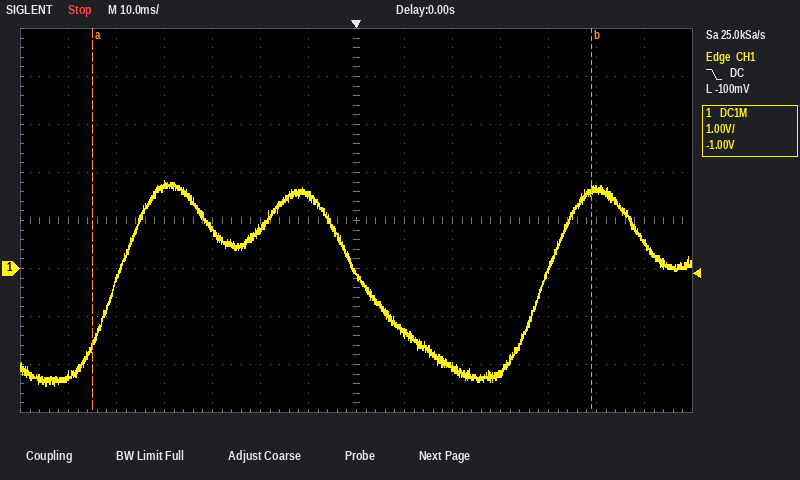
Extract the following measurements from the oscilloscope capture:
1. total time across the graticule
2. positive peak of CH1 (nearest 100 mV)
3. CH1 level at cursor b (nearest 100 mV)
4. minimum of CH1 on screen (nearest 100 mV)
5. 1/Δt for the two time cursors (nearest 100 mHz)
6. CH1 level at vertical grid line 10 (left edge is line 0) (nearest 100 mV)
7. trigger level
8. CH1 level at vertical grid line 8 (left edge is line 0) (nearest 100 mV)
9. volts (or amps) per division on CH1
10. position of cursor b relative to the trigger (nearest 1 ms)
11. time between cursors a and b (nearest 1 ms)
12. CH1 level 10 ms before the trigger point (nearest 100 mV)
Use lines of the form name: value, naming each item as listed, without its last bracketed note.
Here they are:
total time across the graticule: 140 ms
positive peak of CH1: 1.8 V
CH1 level at cursor b: 1.6 V
minimum of CH1 on screen: -2.4 V
1/Δt for the two time cursors: 9.6 Hz
CH1 level at vertical grid line 10 (left edge is line 0): -2.2 V
trigger level: -100 mV
CH1 level at vertical grid line 8 (left edge is line 0): -1.3 V
volts (or amps) per division on CH1: 1 V
position of cursor b relative to the trigger: +49 ms
time between cursors a and b: 104 ms
CH1 level 10 ms before the trigger point: 1.5 V
